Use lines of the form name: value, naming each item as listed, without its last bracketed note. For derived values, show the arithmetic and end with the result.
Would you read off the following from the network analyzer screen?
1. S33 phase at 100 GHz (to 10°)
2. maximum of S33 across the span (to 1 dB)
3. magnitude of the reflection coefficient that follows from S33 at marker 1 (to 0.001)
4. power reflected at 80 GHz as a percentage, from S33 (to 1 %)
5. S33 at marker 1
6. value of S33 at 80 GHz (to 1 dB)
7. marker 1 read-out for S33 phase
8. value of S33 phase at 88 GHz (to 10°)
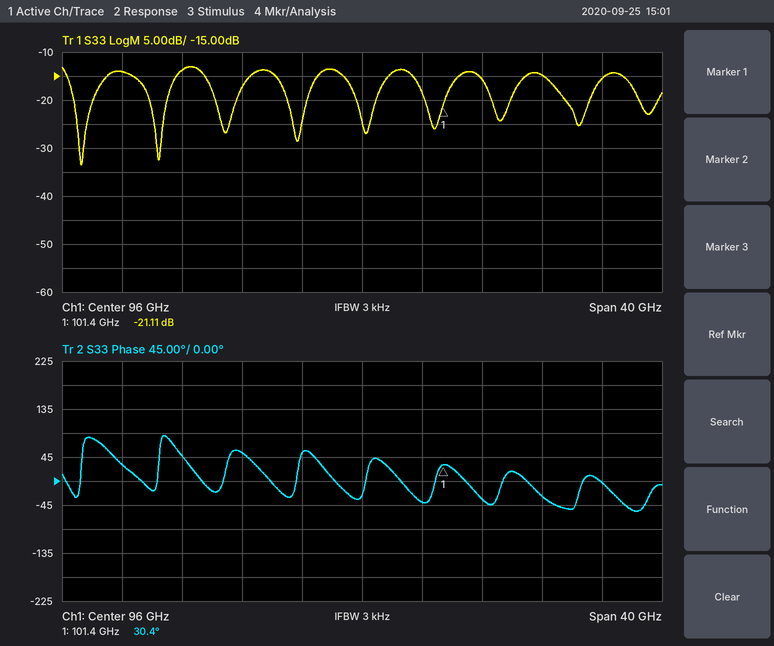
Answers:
S33 phase at 100 GHz: -40°
maximum of S33 across the span: -13 dB
magnitude of the reflection coefficient that follows from S33 at marker 1: 10^(-21.11/20) ≈ 0.088
power reflected at 80 GHz as a percentage, from S33: 10^(-14/10) ≈ 4 %
S33 at marker 1: -21.11 dB
value of S33 at 80 GHz: -14 dB
marker 1 read-out for S33 phase: 30.4°
value of S33 phase at 88 GHz: 50°
